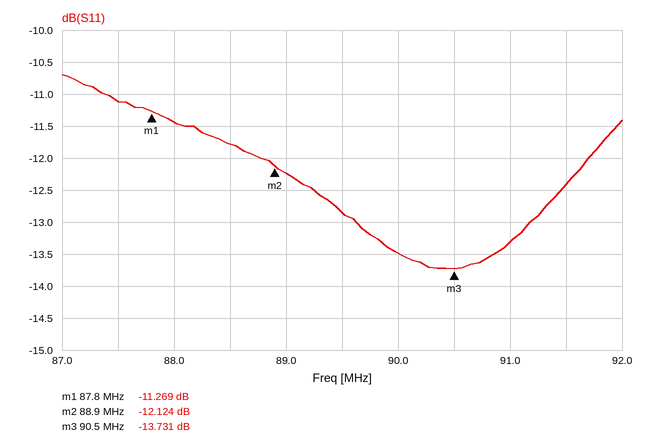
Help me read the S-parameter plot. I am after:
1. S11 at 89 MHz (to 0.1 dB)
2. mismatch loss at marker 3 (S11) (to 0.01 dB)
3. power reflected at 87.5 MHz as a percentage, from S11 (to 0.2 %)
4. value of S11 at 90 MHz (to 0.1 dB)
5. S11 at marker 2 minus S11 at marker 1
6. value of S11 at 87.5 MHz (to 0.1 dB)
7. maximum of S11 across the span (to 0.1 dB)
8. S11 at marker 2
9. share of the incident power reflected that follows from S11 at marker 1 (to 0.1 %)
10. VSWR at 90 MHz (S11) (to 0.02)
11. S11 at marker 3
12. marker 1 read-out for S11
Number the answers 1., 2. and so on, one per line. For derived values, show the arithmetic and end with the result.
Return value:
1. -12.2 dB
2. −10 log10(1 − 10^(-13.731/10)) ≈ 0.19 dB
3. 10^(-11.1/10) ≈ 7.8 %
4. -13.5 dB
5. -12.124 − (-11.269) = -0.855 dB
6. -11.1 dB
7. -10.7 dB
8. -12.124 dB
9. 10^(-11.269/10) ≈ 7.5 %
10. |Γ| = 10^(-13.5/20) = 0.2113; VSWR = (1 + 0.2113)/(1 − 0.2113) ≈ 1.54
11. -13.731 dB
12. -11.269 dB
